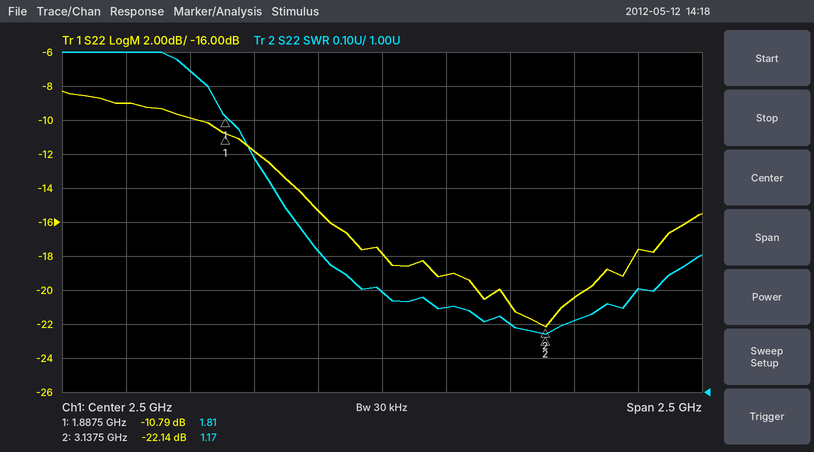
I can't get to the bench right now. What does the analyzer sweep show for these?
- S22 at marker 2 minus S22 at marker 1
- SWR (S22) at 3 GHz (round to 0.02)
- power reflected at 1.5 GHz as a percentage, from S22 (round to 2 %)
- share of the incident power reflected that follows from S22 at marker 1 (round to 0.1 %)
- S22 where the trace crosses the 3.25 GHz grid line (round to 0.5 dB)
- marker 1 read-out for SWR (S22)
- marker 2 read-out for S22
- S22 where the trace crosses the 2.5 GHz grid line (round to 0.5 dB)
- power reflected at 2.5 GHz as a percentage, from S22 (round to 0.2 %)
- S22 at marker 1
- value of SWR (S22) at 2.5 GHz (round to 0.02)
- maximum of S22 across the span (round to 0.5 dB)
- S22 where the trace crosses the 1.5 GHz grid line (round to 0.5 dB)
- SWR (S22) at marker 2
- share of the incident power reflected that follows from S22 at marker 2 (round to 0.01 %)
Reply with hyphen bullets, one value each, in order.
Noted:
- -11.35 dB
- 1.20
- 12 %
- 8.3 %
- -20.5 dB
- 1.81
- -22.14 dB
- -18.0 dB
- 1.6 %
- -10.79 dB
- 1.30
- -8.5 dB
- -9.0 dB
- 1.17
- 0.61 %
